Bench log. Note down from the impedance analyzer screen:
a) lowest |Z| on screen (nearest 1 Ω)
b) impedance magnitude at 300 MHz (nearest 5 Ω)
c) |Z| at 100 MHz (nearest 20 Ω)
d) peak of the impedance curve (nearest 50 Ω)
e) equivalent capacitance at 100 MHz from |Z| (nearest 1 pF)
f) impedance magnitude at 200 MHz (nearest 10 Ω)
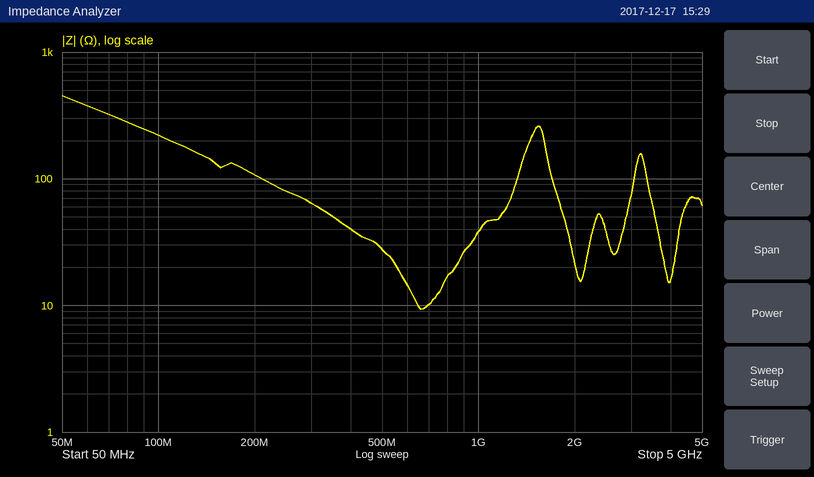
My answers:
9 Ω
65 Ω
220 Ω
450 Ω
7 pF
110 Ω
